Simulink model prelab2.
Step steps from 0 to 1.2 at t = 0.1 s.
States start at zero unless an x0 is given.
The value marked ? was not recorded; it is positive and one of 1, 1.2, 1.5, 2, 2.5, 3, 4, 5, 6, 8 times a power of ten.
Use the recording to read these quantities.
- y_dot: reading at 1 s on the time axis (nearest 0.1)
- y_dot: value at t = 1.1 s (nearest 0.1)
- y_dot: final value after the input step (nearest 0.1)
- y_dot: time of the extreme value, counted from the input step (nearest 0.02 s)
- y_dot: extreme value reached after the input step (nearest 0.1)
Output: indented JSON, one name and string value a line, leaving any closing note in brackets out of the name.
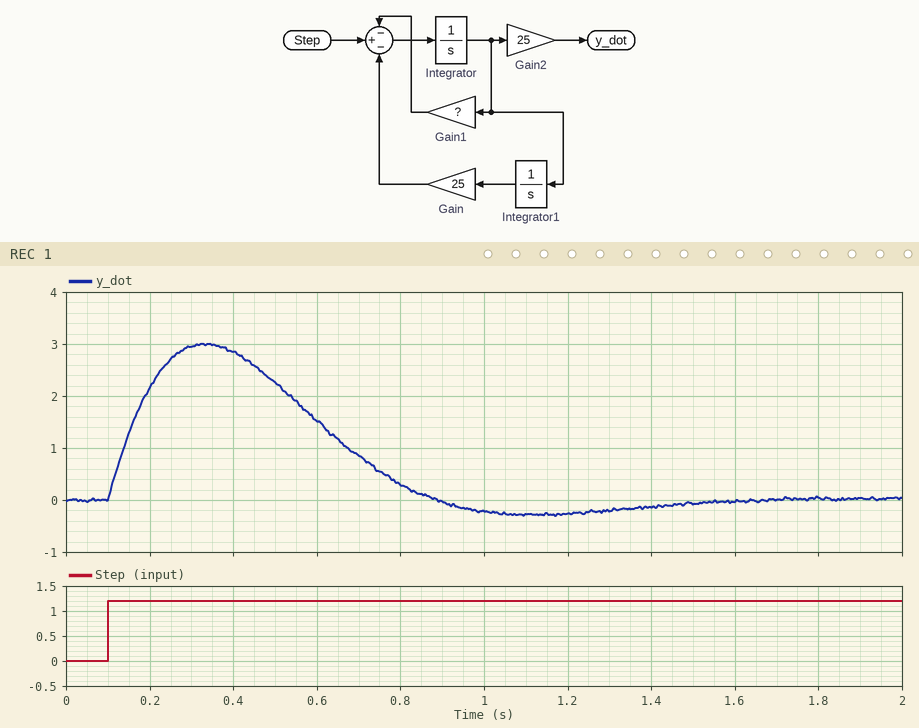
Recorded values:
{
  "y_dot: reading at 1 s on the time axis": "-0.2",
  "y_dot: value at t = 1.1 s": "-0.3",
  "y_dot: final value after the input step": "0.0",
  "y_dot: time of the extreme value, counted from the input step": "0.24 s",
  "y_dot: extreme value reached after the input step": "3.0"
}
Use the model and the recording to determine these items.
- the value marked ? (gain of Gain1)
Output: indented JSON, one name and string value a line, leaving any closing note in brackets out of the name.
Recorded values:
{
  "the value marked ?": "6"
}
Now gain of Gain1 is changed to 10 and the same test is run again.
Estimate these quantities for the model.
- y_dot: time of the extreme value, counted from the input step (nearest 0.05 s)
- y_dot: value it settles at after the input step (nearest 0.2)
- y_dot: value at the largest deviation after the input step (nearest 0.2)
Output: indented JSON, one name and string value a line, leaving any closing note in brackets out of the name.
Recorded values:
{
  "y_dot: time of the extreme value, counted from the input step": "0.20 s",
  "y_dot: value it settles at after the input step": "0.0",
  "y_dot: value at the largest deviation after the input step": "2.2"
}
